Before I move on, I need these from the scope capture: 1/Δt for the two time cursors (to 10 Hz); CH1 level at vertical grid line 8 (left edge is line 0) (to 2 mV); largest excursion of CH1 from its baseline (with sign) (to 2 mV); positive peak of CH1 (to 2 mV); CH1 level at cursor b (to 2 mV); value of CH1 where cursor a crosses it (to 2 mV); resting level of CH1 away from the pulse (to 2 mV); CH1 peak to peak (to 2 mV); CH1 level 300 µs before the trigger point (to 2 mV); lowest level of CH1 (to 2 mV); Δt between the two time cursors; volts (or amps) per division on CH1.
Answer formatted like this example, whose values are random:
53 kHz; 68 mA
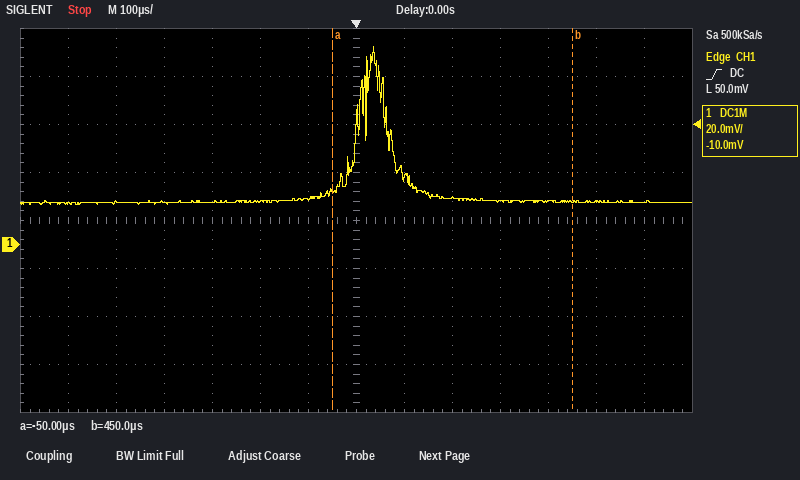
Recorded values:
2.00 kHz; 28 mV; +64 mV; 82 mV; 18 mV; 22 mV; 18 mV; 66 mV; 18 mV; 16 mV; 500 µs; 20 mV
